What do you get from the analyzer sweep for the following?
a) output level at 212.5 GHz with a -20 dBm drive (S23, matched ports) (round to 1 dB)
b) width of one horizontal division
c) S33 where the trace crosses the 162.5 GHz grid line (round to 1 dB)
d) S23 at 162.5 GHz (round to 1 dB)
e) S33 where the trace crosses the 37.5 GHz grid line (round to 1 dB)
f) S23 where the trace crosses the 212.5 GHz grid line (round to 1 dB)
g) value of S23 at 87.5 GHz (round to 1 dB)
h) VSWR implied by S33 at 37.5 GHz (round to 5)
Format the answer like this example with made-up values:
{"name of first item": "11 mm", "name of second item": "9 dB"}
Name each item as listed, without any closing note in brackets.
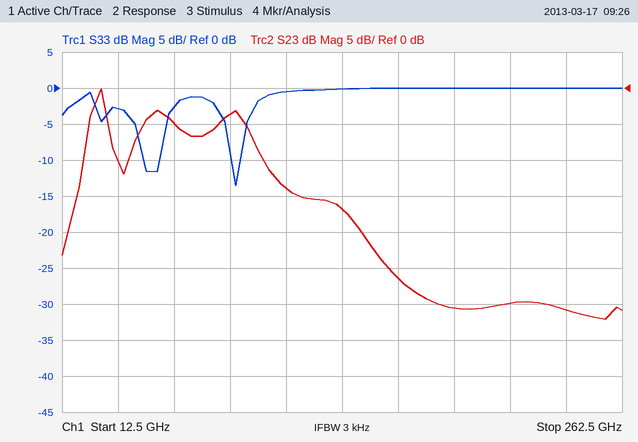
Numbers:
{"output level at 212.5 GHz with a -20 dBm drive (S23, matched ports)": "-50 dBm", "width of one horizontal division": "25 GHz", "S33 where the trace crosses the 162.5 GHz grid line": "0 dB", "S23 at 162.5 GHz": "-26 dB", "S33 where the trace crosses the 37.5 GHz grid line": "-3 dB", "S23 where the trace crosses the 212.5 GHz grid line": "-30 dB", "value of S23 at 87.5 GHz": "-4 dB", "VSWR implied by S33 at 37.5 GHz": "5"}
